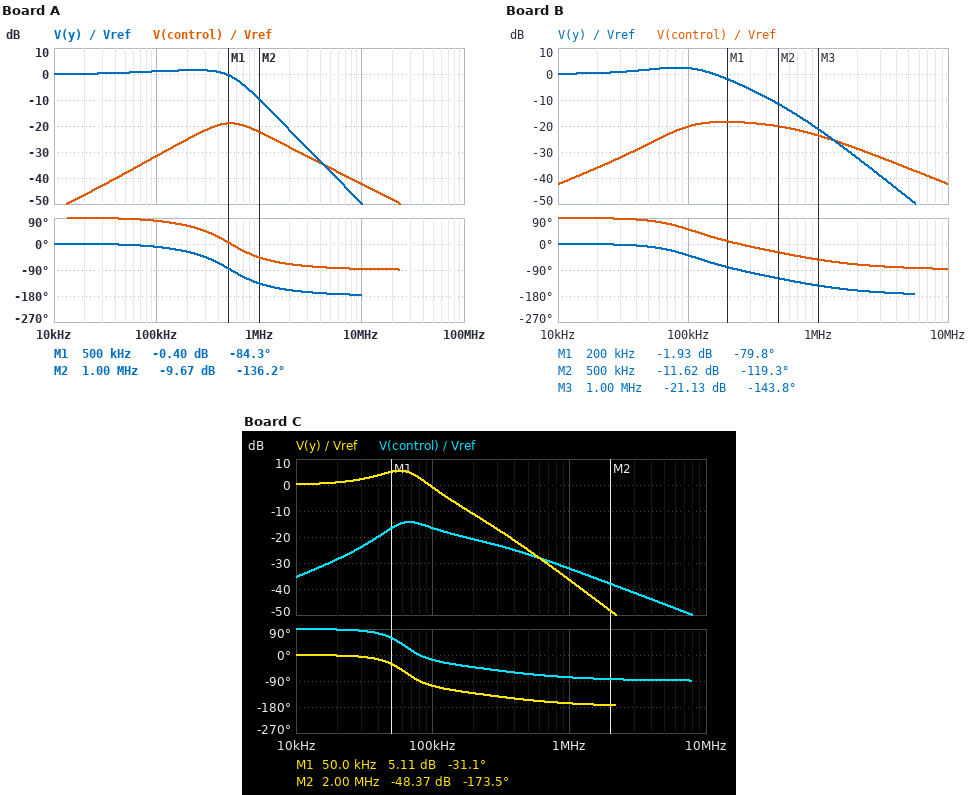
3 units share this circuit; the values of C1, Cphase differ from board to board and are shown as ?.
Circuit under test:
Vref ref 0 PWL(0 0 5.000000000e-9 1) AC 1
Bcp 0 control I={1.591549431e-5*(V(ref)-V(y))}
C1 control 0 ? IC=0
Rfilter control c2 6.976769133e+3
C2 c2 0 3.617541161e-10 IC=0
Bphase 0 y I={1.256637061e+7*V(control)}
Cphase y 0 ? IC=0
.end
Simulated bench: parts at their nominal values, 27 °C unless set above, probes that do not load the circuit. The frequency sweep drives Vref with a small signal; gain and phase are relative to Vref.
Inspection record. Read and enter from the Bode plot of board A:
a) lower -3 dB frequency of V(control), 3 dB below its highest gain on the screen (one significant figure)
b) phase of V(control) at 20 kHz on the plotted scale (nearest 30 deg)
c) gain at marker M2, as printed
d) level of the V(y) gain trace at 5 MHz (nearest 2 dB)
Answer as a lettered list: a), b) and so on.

a) 300 kHz
b) 90 deg
c) -9.67 dB
d) -38 dB
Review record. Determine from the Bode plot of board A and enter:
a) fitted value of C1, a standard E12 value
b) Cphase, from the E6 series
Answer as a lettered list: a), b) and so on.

a) 33 pF
b) 470 mF
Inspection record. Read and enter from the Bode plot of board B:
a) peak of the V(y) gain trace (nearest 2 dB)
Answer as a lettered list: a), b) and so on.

a) 2 dB
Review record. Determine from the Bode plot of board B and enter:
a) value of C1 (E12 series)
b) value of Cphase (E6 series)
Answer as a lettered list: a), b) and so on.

a) 33 pF
b) 1.5 F
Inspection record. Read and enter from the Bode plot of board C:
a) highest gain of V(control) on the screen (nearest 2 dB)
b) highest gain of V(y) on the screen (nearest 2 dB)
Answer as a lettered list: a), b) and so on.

a) -14 dB
b) 6 dB
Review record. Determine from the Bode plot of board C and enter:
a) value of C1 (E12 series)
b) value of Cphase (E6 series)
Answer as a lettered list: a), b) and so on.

a) 100 pF
b) 3.3 F
